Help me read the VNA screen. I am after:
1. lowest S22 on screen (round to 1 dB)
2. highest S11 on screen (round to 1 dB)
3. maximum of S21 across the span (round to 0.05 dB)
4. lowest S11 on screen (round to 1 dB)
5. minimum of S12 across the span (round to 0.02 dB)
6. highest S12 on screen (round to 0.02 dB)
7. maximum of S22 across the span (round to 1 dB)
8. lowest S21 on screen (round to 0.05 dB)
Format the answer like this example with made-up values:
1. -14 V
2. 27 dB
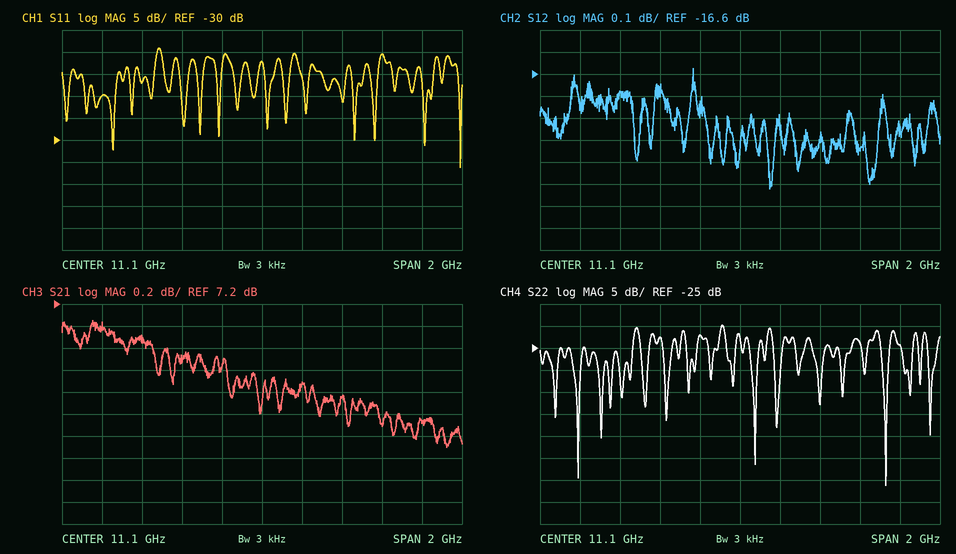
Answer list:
1. -56 dB
2. -9 dB
3. 7.05 dB
4. -36 dB
5. -17.12 dB
6. -16.58 dB
7. -20 dB
8. 5.90 dB
